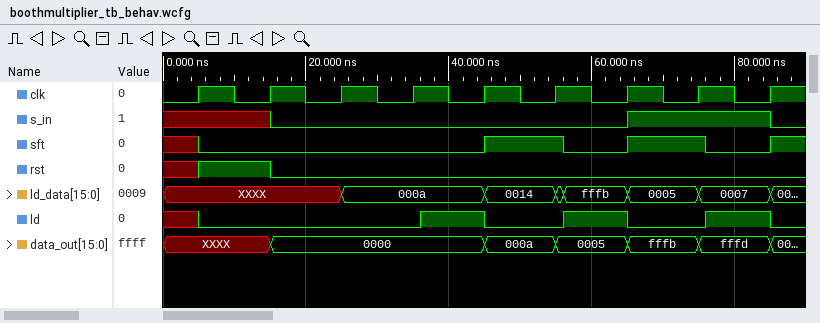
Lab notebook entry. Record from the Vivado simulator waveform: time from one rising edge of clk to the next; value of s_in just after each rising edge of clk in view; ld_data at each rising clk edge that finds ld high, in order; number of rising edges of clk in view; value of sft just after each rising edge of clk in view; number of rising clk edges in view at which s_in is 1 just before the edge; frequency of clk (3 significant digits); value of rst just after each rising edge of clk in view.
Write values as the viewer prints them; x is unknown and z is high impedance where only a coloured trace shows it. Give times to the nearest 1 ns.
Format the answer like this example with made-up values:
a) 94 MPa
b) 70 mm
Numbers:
a) 10 ns
b) x 0 0 0 0 0 1 1 0
c) 000a, fffb, 0007
d) 9
e) 0 0 0 0 1 1 1 1 1
f) 2
g) 100 MHz
h) 1 0 0 0 0 0 0 0 0
